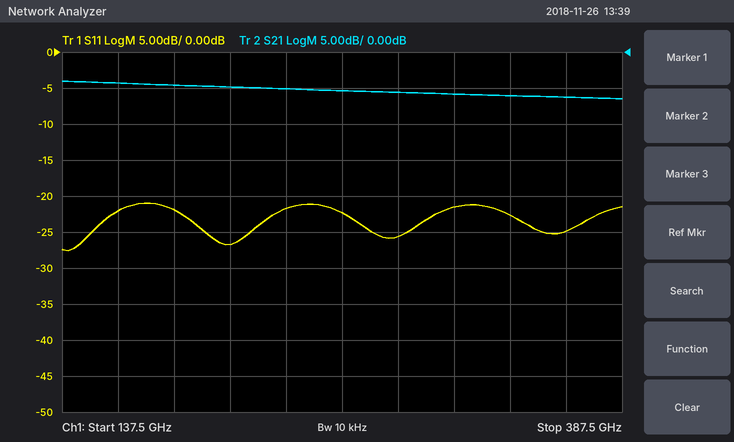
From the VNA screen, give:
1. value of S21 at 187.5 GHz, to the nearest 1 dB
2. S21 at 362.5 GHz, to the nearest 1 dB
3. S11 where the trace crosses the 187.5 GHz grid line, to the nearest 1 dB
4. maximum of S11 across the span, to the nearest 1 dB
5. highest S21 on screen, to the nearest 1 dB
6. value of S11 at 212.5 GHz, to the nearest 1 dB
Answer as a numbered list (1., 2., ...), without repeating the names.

1. -5 dB
2. -6 dB
3. -22 dB
4. -21 dB
5. -4 dB
6. -27 dB
